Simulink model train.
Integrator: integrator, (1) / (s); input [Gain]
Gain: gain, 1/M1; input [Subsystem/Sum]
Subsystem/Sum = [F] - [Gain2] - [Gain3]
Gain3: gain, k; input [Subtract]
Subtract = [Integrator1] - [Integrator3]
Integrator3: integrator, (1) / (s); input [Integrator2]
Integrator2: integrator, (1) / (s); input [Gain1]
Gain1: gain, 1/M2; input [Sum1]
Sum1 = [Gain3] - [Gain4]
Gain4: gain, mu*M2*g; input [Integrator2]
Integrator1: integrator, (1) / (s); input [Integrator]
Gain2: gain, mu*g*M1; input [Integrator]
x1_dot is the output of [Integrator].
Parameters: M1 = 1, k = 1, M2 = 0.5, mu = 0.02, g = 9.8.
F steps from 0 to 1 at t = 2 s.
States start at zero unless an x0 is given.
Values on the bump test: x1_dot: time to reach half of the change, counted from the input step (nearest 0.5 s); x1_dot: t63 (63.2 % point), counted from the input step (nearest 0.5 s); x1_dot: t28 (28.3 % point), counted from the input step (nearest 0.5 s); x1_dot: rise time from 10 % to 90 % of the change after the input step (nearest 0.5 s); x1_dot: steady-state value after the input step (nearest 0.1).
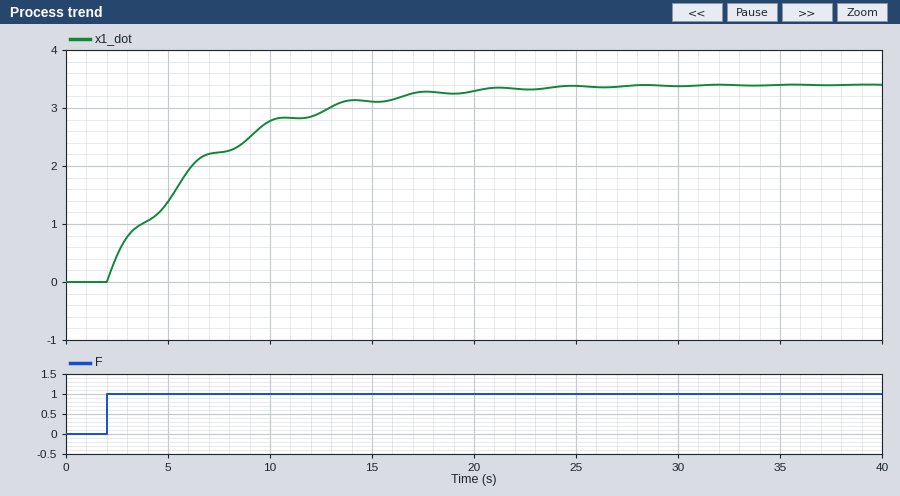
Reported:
3.5 s
4.5 s
1.5 s
11.0 s
3.4
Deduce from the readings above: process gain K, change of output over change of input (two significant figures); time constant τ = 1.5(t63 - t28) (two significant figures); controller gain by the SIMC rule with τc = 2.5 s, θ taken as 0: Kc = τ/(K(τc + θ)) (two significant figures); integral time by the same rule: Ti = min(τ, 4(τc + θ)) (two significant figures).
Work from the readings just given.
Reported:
3.4
4.5 s
0.53
4.5 s
